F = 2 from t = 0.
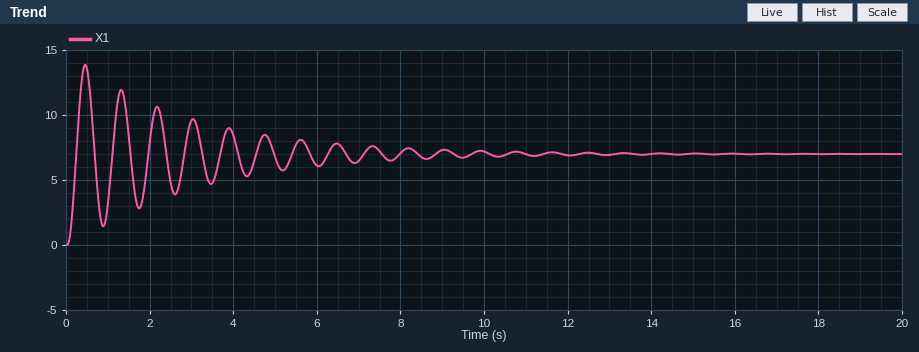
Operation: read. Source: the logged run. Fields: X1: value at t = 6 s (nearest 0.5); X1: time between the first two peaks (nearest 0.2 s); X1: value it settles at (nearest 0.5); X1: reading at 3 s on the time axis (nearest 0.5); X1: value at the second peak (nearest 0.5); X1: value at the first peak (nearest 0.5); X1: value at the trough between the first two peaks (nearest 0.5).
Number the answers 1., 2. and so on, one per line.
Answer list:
1. 6.0
2. 0.8 s
3. 7.0
4. 9.5
5. 12.0
6. 14.0
7. 1.5
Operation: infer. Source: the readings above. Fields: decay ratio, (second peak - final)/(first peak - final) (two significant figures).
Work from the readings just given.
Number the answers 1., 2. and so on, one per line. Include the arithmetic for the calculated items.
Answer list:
1. (12 - 7) / (14 - 7) = 0.71
